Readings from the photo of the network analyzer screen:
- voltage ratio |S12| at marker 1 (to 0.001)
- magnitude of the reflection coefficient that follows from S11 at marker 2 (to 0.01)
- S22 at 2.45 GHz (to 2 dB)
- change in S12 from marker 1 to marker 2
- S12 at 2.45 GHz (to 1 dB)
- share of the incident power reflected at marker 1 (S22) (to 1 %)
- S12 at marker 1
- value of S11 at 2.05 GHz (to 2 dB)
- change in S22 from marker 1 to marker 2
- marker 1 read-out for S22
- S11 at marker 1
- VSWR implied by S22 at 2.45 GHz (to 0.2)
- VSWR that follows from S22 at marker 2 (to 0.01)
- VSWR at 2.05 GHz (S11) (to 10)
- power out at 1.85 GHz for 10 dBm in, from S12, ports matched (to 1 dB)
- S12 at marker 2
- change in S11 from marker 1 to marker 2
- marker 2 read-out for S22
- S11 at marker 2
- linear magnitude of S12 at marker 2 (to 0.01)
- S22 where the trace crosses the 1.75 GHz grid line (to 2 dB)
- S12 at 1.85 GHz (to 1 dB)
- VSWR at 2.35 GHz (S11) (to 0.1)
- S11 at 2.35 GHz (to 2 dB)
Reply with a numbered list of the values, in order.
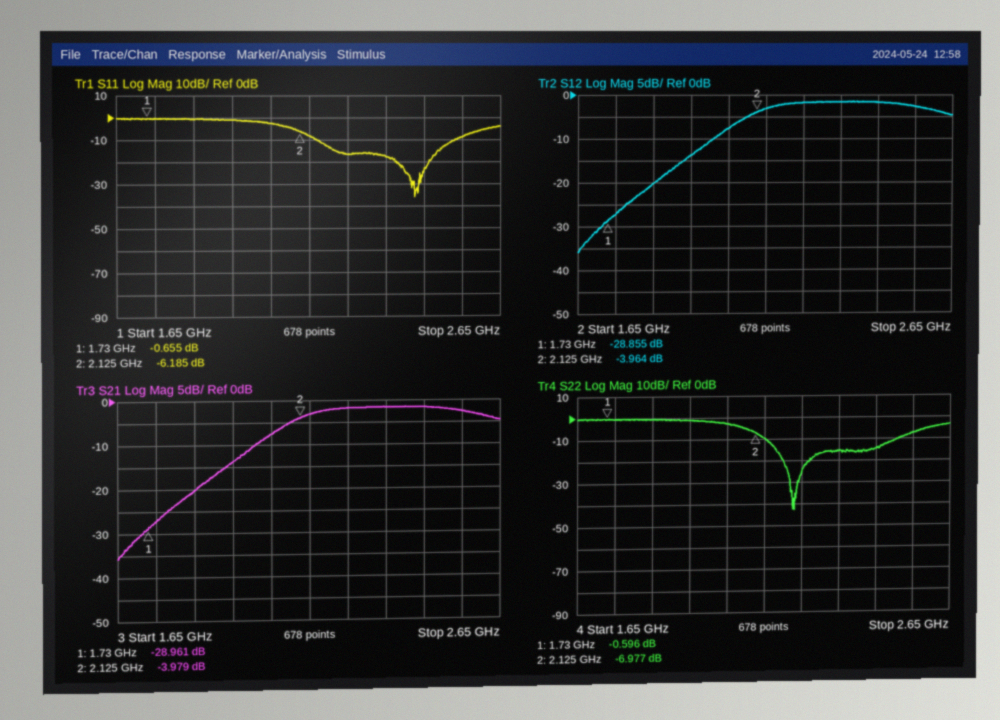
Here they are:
1. 0.036
2. 0.49
3. -14 dB
4. 24.891 dB
5. -2 dB
6. 87 %
7. -28.855 dB
8. -2 dB
9. -6.381 dB
10. -0.596 dB
11. -0.655 dB
12. 1.4
13. 2.62
14. 10
15. -10 dBm
16. -3.964 dB
17. -5.530 dB
18. -6.977 dB
19. -6.185 dB
20. 0.63
21. 0 dB
22. -20 dB
23. 1.3
24. -18 dB
